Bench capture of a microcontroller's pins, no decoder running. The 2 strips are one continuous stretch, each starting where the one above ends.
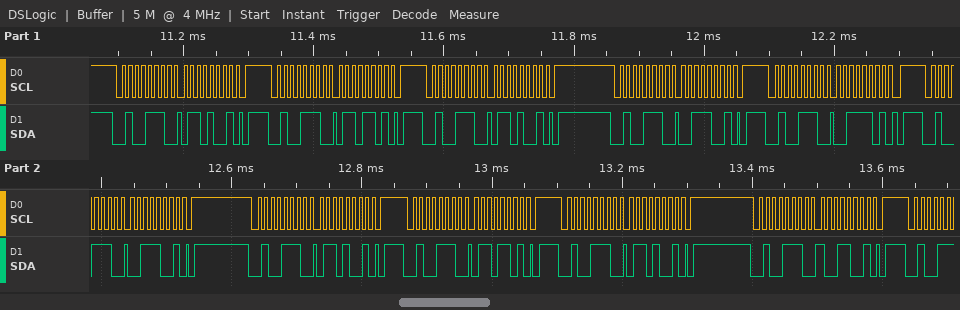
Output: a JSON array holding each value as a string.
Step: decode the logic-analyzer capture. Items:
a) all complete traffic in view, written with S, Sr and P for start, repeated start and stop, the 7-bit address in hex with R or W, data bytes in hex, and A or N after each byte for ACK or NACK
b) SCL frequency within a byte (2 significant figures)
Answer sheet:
["S 27W A 69 A P S 27W A 6D A P S 27W A 69 A P S 27W A 39 A P S 27W A 3D A P S 27W A 39 A P S 27W A 69 A P S 27W A 6D A P S 27W A 69 A P S 27W A 99 A P", "100 kHz"]
